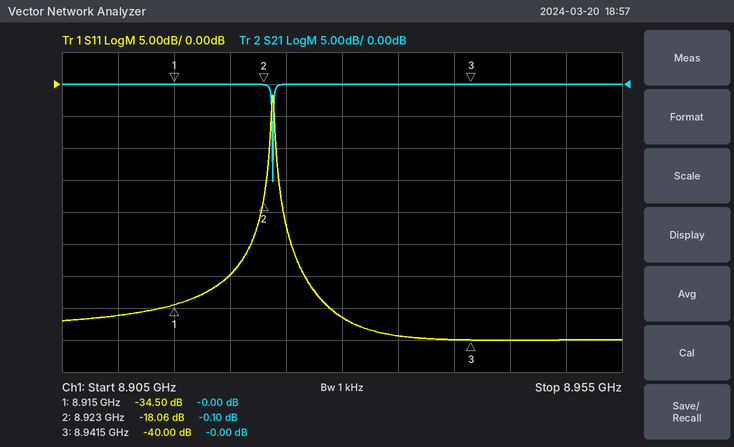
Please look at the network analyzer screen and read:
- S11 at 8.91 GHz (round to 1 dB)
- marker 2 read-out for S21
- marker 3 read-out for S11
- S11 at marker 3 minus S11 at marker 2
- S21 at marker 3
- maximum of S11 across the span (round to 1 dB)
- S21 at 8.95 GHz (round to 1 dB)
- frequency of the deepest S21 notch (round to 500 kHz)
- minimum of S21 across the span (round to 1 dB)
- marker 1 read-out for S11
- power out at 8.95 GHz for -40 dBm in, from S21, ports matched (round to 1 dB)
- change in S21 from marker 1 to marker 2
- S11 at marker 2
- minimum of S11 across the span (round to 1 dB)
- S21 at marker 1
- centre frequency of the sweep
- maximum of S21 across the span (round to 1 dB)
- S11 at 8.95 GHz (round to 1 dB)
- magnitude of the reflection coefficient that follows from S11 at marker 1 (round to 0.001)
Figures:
-36 dB
-0.10 dB
-40.00 dB
-21.94 dB
-0.00 dB
-2 dB
0 dB
8.9240 GHz
-15 dB
-34.50 dB
-40 dBm
-0.10 dB
-18.06 dB
-40 dB
-0.00 dB
8.93 GHz
0 dB
-40 dB
0.019
